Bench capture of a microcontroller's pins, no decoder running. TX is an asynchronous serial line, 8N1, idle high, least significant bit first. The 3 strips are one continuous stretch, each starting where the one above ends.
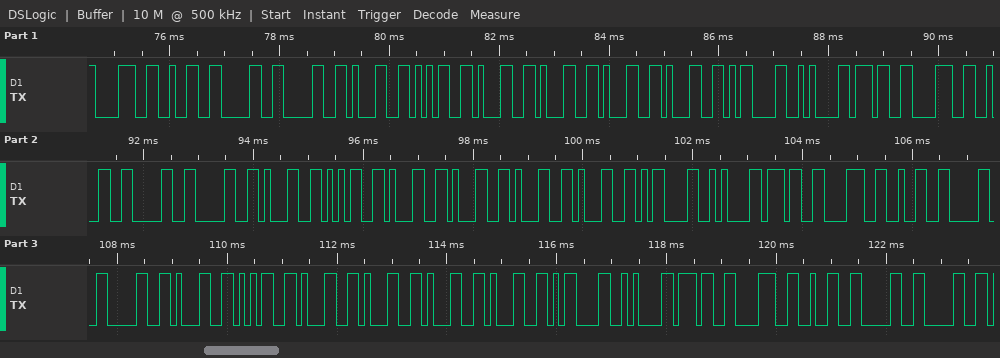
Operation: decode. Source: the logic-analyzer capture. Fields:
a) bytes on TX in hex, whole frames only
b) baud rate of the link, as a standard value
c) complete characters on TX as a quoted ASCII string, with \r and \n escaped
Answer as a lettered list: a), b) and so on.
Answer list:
a) 38 32 30 30 31 35 31 31 31 31 0D 0A 37 38 32 30 30 31 35 31 31 31 31 0D 0A 37 38 32 30 30 31 35 31 31 31 31 0D 0A 37 38 32 30 30
b) 9600 baud
c) "8200151111\r\n78200151111\r\n78200151111\r\n78200"
